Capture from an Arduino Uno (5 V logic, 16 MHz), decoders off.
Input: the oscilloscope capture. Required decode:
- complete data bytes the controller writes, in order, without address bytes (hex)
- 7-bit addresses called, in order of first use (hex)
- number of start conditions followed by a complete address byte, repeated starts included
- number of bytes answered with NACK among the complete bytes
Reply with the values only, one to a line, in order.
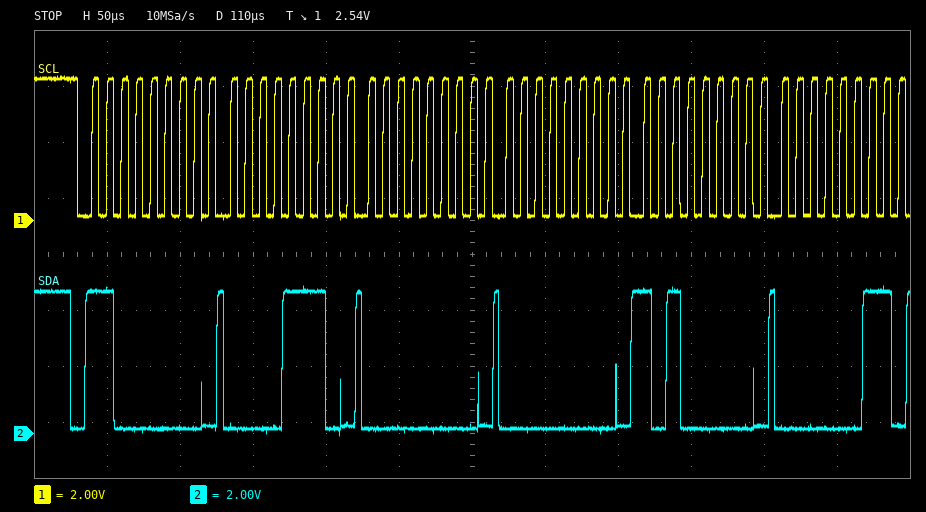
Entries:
0E 00 00 A0 03
0x60
1
0
